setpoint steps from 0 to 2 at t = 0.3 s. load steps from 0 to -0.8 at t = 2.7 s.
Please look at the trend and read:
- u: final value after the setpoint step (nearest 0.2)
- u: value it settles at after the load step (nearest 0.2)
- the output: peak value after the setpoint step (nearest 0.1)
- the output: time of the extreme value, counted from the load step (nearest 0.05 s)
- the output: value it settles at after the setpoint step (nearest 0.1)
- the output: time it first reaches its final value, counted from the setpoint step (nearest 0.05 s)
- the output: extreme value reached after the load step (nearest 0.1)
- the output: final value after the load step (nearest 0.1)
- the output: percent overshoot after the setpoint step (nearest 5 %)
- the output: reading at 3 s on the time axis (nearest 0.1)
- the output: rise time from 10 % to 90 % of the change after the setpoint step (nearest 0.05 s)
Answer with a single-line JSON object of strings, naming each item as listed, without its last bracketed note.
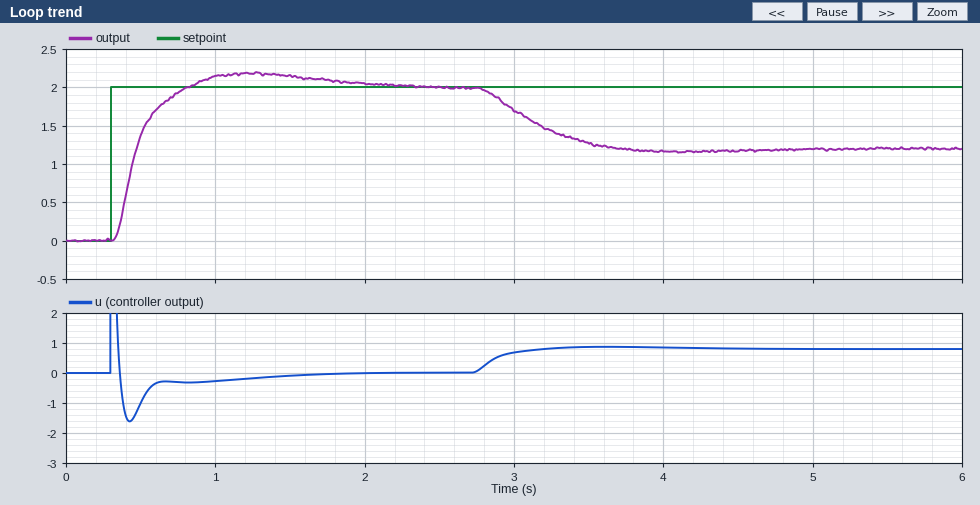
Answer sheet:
{"u: final value after the setpoint step": "0.0", "u: value it settles at after the load step": "0.8", "the output: peak value after the setpoint step": "2.2", "the output: time of the extreme value, counted from the load step": "1.40 s", "the output: value it settles at after the setpoint step": "2.0", "the output: time it first reaches its final value, counted from the setpoint step": "0.50 s", "the output: extreme value reached after the load step": "1.2", "the output: final value after the load step": "1.2", "the output: percent overshoot after the setpoint step": "10 %", "the output: reading at 3 s on the time axis": "1.7", "the output: rise time from 10 % to 90 % of the change after the setpoint step": "0.30 s"}
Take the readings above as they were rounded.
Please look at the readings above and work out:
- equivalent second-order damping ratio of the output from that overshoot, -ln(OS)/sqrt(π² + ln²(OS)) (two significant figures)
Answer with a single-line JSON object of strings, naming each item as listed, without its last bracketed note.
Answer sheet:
{"equivalent second-order damping ratio of the output from that overshoot, -ln(OS)/sqrt(π² + ln²(OS))": "0.59"}
